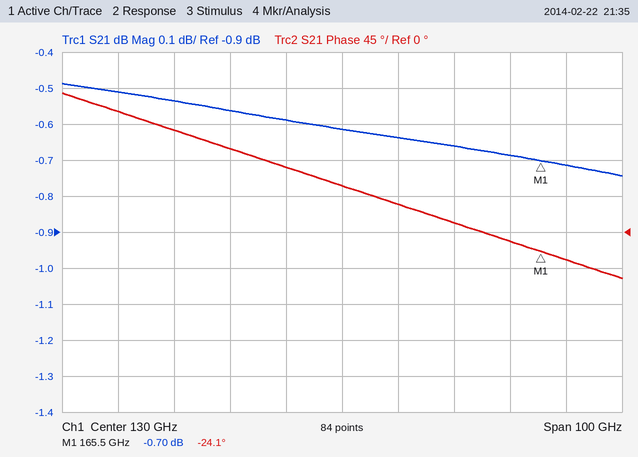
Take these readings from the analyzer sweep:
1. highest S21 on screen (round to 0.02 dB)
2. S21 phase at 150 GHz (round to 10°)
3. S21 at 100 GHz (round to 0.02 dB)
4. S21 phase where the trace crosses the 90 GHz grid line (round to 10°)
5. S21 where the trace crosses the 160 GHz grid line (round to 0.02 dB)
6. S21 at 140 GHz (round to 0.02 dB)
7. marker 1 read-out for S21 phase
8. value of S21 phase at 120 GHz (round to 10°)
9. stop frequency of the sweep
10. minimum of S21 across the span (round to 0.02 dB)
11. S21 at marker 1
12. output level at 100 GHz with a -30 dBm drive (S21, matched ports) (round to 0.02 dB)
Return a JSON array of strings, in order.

["-0.48 dB", "10°", "-0.54 dB", "150°", "-0.68 dB", "-0.64 dB", "-24.1°", "80°", "180 GHz", "-0.74 dB", "-0.70 dB", "-30.54 dBm"]
